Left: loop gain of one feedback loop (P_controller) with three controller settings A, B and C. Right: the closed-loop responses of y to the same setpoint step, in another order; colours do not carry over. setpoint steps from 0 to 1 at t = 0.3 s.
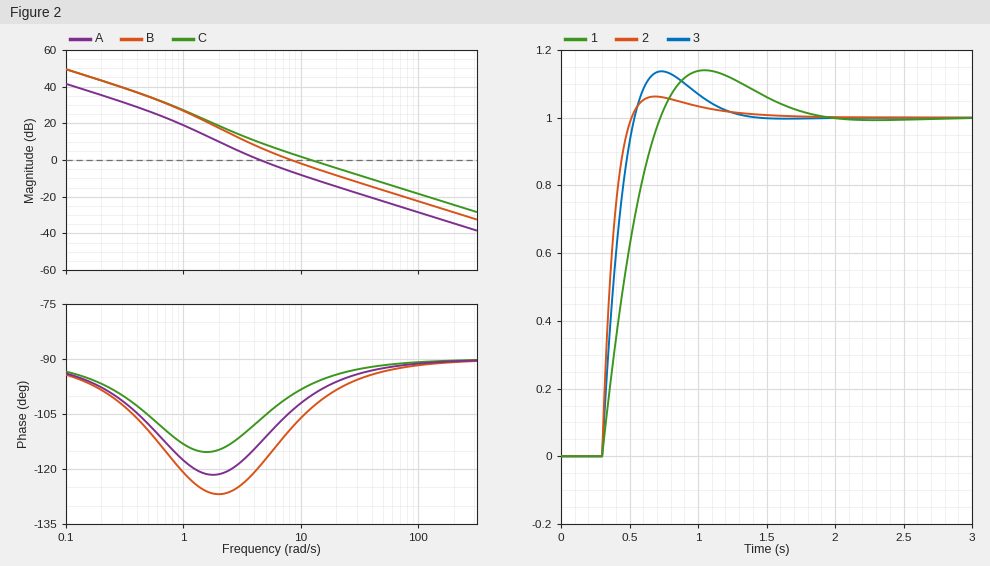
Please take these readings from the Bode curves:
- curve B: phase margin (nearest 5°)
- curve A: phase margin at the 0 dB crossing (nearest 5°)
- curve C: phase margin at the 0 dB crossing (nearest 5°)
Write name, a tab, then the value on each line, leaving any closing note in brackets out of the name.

curve B: phase margin	70°
curve A: phase margin at the 0 dB crossing	65°
curve C: phase margin at the 0 dB crossing	85°
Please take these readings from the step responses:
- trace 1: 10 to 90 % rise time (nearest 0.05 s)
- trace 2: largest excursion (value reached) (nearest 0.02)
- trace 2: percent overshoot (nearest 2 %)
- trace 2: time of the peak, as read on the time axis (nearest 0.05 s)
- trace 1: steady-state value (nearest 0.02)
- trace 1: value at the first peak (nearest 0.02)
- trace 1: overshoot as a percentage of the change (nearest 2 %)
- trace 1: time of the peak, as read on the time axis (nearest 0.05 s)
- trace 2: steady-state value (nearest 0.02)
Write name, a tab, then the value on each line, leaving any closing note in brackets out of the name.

trace 1: 10 to 90 % rise time	0.30 s
trace 2: largest excursion (value reached)	1.06
trace 2: percent overshoot	6 %
trace 2: time of the peak, as read on the time axis	0.70 s
trace 1: steady-state value	1.00
trace 1: value at the first peak	1.14
trace 1: overshoot as a percentage of the change	14 %
trace 1: time of the peak, as read on the time axis	1.05 s
trace 2: steady-state value	1.00
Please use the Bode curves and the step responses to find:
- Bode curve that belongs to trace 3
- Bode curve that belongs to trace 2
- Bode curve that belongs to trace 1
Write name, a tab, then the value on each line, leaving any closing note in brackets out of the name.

Bode curve that belongs to trace 3	B
Bode curve that belongs to trace 2	C
Bode curve that belongs to trace 1	A
